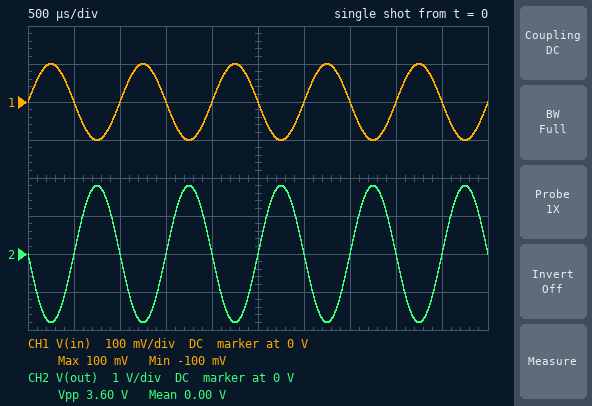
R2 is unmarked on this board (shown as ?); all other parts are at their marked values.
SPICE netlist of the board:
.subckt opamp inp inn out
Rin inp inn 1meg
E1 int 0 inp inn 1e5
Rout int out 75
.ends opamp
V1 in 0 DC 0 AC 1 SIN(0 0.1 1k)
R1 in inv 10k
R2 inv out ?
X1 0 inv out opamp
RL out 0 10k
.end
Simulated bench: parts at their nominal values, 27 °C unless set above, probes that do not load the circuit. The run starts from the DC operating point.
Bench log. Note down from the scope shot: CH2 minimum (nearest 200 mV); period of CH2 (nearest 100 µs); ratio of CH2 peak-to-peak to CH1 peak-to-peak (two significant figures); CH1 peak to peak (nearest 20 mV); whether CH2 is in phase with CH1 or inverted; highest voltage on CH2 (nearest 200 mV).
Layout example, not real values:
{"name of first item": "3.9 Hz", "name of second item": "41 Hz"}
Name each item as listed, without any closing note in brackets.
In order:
{"CH2 minimum": "-1.8 V", "period of CH2": "1.0 ms", "ratio of CH2 peak-to-peak to CH1 peak-to-peak": "18", "CH1 peak to peak": "200 mV", "whether CH2 is in phase with CH1 or inverted": "inverted", "highest voltage on CH2": "1.8 V"}
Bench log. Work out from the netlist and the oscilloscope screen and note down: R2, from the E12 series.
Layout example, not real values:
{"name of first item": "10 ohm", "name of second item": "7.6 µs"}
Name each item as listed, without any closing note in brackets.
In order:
{"R2, from the E12 series": "180 kΩ"}
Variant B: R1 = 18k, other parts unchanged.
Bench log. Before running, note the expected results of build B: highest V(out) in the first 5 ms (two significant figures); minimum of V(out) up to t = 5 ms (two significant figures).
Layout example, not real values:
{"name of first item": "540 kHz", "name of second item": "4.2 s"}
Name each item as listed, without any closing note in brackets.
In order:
{"highest V(out) in the first 5 ms": "1.0 V", "minimum of V(out) up to t = 5 ms": "-1.0 V"}
